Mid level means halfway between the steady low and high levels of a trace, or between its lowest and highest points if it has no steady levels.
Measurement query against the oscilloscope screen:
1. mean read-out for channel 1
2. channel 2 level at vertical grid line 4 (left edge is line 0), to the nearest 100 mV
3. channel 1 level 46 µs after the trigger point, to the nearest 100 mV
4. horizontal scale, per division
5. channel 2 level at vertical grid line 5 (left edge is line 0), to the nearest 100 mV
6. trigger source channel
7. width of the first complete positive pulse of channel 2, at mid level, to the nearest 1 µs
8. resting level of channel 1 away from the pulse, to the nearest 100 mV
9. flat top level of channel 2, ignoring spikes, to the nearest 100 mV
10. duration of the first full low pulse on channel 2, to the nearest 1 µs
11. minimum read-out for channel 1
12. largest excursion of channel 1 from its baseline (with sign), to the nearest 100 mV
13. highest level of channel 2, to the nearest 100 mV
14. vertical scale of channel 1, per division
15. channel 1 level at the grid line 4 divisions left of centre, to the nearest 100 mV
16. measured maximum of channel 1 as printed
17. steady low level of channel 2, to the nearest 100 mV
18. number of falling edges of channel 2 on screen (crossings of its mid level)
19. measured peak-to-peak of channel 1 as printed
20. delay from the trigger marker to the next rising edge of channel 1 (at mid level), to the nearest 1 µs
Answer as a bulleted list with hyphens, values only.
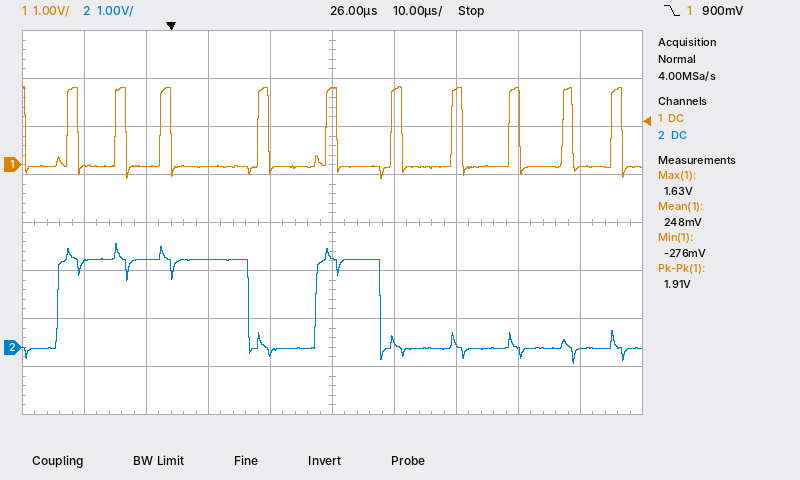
- 248 mV
- -100 mV
- 1.6 V
- 10 µs
- 1.9 V
- channel 1
- 31 µs
- 0.0 V
- 1.8 V
- 11 µs
- -276 mV
- +1.7 V
- 2.2 V
- 1 V
- 0.0 V
- 1.63 V
- 0.0 V
- 2
- 1.91 V
- 14 µs
